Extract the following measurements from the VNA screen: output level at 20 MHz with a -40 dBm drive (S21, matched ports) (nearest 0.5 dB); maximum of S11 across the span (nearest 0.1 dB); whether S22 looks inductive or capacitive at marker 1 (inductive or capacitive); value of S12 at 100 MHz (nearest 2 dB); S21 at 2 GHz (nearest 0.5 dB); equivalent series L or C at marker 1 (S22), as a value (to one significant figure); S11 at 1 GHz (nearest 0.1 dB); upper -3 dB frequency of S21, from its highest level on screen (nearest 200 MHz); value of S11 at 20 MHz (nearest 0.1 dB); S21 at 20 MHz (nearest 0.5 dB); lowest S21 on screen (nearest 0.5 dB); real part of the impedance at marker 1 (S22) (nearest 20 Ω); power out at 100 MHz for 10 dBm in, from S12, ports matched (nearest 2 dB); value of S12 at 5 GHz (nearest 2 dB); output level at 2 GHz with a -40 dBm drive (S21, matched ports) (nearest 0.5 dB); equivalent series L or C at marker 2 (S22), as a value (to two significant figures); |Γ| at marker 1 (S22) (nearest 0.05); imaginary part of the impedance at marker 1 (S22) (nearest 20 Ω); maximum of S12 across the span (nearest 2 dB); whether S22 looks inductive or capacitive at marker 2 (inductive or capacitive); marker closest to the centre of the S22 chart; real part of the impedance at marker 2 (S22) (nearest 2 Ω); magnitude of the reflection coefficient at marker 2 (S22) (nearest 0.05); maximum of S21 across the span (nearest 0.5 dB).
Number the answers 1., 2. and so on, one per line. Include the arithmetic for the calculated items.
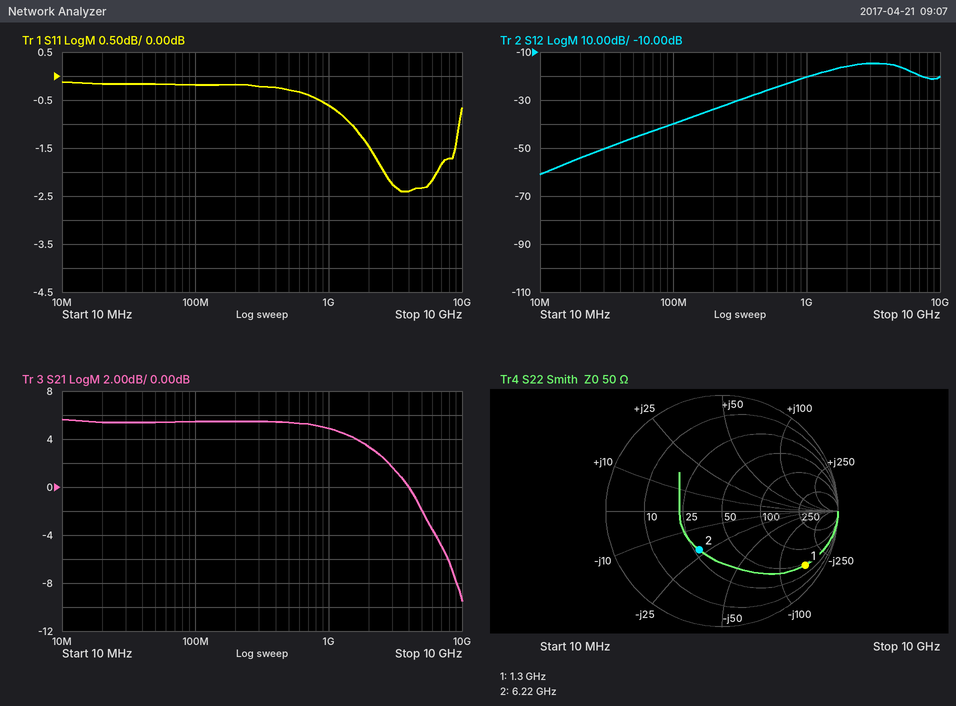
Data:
1. -40 dBm + (5.5 dB) = -34.5 dBm
2. -0.1 dB
3. capacitive
4. -40 dB
5. 3.5 dB
6. C = 1/(2π × 1.3 GHz × 160 Ω) ≈ 765 fF, so 800 fF to one significant figure
7. -0.6 dB
8. 2.4 GHz
9. -0.2 dB
10. 5.5 dB
11. -9.5 dB
12. 40 Ω
13. 10 dBm + (-40 dB) = -30 dBm
14. -16 dB
15. -40 dBm + (3.5 dB) = -36.5 dBm
16. C = 1/(2π × 6.22 GHz × 22 Ω) ≈ 1.2 pF
17. 0.85
18. -160 Ω
19. -14 dB
20. capacitive
21. marker 2
22. 28 Ω
23. 0.40
24. 5.5 dB
